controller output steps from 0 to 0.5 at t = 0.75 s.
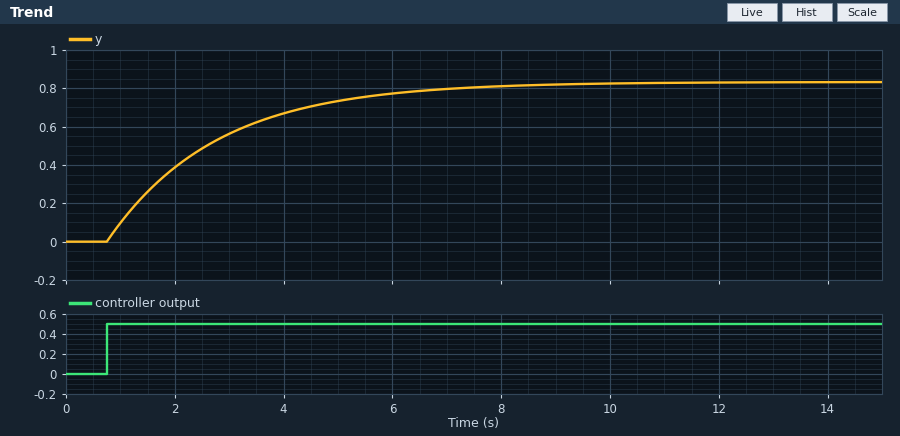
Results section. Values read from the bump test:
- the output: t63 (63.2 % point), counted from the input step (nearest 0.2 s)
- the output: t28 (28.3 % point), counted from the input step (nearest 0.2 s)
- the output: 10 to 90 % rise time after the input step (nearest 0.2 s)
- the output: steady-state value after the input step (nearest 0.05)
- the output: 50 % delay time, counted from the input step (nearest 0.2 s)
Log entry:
2.0 s
0.6 s
4.4 s
0.85
1.4 s
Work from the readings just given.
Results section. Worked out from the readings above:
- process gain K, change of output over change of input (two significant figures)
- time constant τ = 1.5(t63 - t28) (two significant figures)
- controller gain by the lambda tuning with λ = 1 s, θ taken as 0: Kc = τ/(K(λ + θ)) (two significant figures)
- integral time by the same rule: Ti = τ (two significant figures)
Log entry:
1.7
2.1 s
1.2
2.1 s
